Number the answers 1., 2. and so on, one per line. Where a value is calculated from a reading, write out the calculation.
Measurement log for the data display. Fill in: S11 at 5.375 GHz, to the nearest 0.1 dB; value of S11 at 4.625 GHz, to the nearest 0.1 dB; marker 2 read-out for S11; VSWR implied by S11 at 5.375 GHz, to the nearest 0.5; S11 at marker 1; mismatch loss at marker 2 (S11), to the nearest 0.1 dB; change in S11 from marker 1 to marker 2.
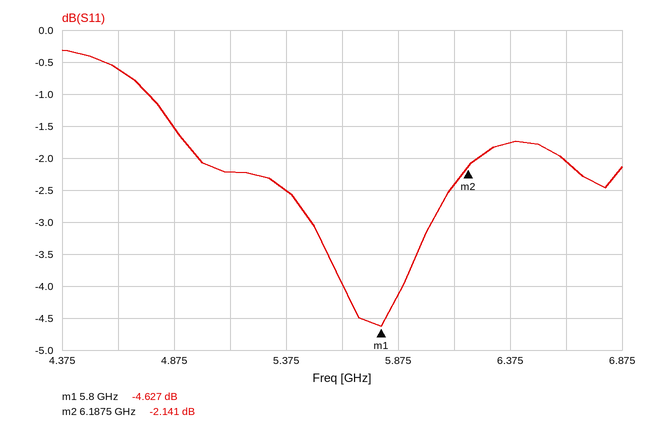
1. -2.5 dB
2. -0.6 dB
3. -2.141 dB
4. |Γ| = 10^(-2.5/20) = 0.7499; VSWR = (1 + 0.7499)/(1 − 0.7499) ≈ 7.0
5. -4.627 dB
6. −10 log10(1 − 10^(-2.141/10)) ≈ 4.1 dB
7. -2.141 − (-4.627) = 2.486 dB
